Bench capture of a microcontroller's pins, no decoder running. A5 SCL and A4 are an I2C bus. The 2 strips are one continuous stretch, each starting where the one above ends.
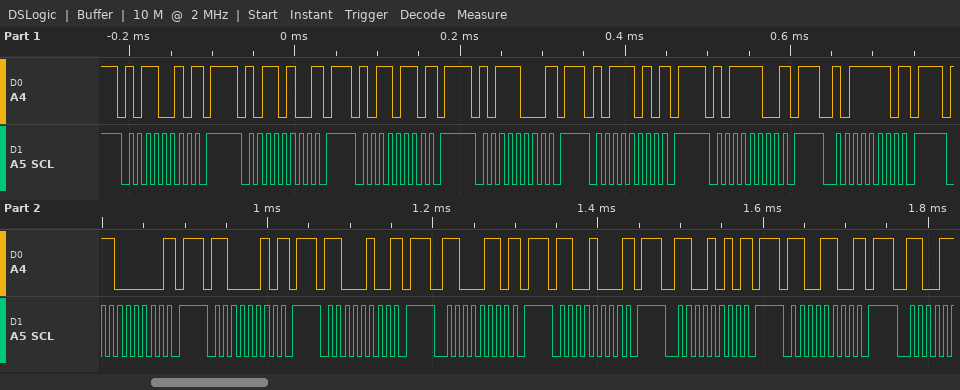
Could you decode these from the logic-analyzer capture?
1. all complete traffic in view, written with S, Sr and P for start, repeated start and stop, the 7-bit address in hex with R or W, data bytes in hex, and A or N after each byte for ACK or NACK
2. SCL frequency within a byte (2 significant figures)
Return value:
S 59W N P S 5AW N P S 5BW N P S 5CW N P S 5DW N P S 5EW N P S 5FW N P S 60W N P S 61W N P S 62W N P S 63W N P S 64W N P S 65W N P S 66W N P
100 kHz
